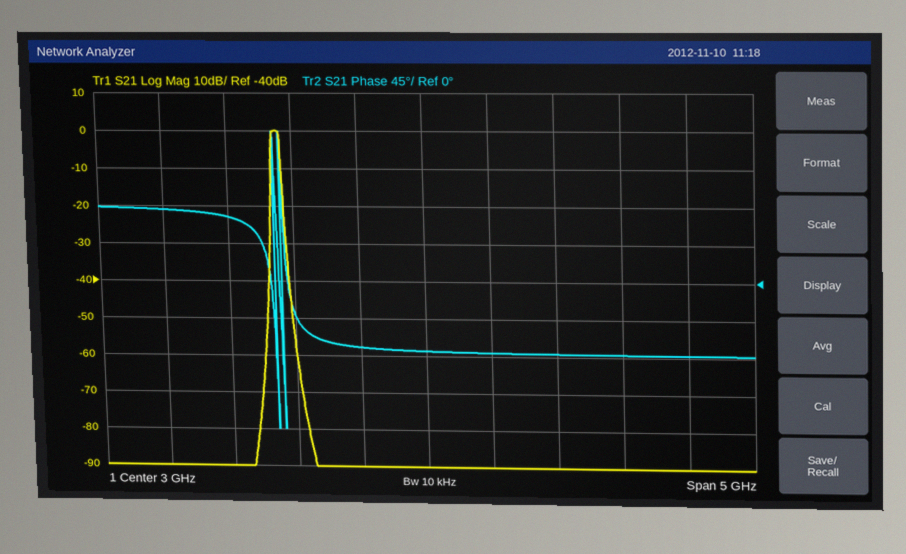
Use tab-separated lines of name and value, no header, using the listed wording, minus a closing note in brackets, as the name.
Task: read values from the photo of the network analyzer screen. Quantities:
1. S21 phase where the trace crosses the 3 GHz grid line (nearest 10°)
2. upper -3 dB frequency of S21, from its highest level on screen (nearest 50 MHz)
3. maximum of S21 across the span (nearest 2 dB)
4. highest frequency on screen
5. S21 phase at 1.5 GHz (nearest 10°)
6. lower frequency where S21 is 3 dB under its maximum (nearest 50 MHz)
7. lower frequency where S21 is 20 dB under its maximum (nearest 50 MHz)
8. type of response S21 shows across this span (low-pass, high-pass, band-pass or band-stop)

S21 phase where the trace crosses the 3 GHz grid line	-80°
upper -3 dB frequency of S21, from its highest level on screen	1.90 GHz
maximum of S21 across the span	0 dB
highest frequency on screen	5.5 GHz
S21 phase at 1.5 GHz	80°
lower frequency where S21 is 3 dB under its maximum	1.85 GHz
lower frequency where S21 is 20 dB under its maximum	1.85 GHz
type of response S21 shows across this span	band-pass
